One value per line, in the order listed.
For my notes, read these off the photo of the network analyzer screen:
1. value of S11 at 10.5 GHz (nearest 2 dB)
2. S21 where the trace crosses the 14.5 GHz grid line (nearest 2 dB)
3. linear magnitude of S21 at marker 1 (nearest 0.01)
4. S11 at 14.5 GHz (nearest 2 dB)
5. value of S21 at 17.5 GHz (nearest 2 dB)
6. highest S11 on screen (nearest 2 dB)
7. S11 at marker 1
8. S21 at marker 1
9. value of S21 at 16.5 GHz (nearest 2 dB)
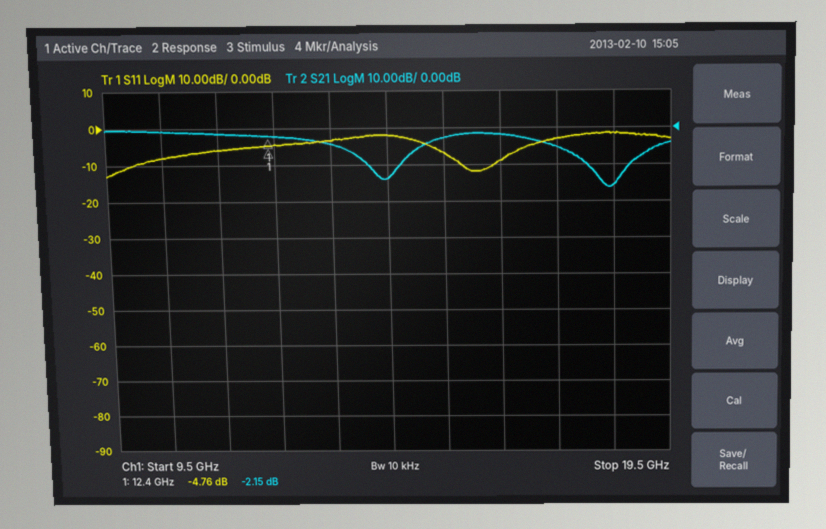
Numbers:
-8 dB
-14 dB
0.78
-2 dB
-6 dB
-2 dB
-4.76 dB
-2.15 dB
-2 dB
